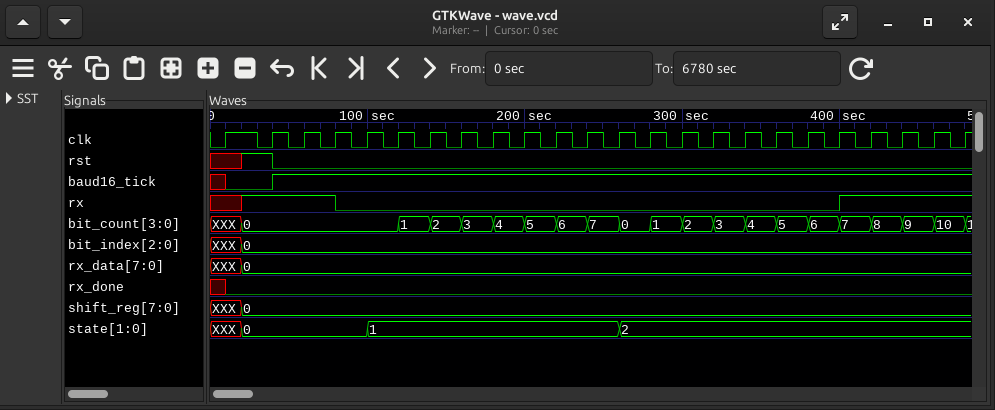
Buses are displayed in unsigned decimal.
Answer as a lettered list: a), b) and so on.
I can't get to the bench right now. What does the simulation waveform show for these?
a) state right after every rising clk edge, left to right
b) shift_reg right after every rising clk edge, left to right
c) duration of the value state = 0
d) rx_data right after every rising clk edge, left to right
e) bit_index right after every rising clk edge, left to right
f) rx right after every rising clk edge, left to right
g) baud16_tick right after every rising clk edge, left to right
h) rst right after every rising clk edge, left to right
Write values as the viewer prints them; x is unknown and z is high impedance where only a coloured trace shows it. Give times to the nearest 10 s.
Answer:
a) XXX, 0, 0, 0, 1, 1, 1, 1, 1, 1, 1, 1, 2, 2, 2, 2, 2, 2, 2, 2, 2, 2, 2, 2
b) XXX, 0, 0, 0, 0, 0, 0, 0, 0, 0, 0, 0, 0, 0, 0, 0, 0, 0, 0, 0, 0, 0, 0, 0
c) 80 s
d) XXX, 0, 0, 0, 0, 0, 0, 0, 0, 0, 0, 0, 0, 0, 0, 0, 0, 0, 0, 0, 0, 0, 0, 0
e) XXX, 0, 0, 0, 0, 0, 0, 0, 0, 0, 0, 0, 0, 0, 0, 0, 0, 0, 0, 0, 0, 0, 0, 0
f) x 1 1 0 0 0 0 0 0 0 0 0 0 0 0 0 0 0 0 1 1 1 1 1
g) 0 1 1 1 1 1 1 1 1 1 1 1 1 1 1 1 1 1 1 1 1 1 1 1
h) x 0 0 0 0 0 0 0 0 0 0 0 0 0 0 0 0 0 0 0 0 0 0 0
